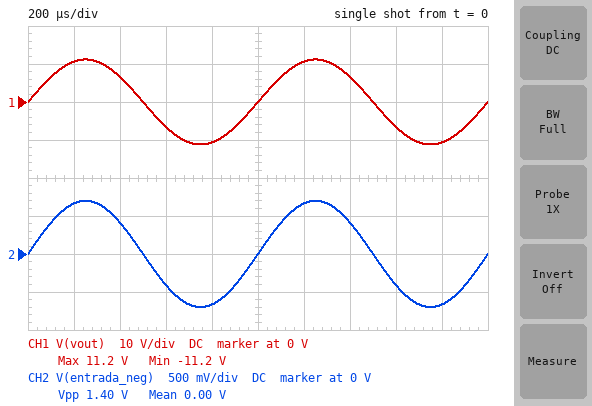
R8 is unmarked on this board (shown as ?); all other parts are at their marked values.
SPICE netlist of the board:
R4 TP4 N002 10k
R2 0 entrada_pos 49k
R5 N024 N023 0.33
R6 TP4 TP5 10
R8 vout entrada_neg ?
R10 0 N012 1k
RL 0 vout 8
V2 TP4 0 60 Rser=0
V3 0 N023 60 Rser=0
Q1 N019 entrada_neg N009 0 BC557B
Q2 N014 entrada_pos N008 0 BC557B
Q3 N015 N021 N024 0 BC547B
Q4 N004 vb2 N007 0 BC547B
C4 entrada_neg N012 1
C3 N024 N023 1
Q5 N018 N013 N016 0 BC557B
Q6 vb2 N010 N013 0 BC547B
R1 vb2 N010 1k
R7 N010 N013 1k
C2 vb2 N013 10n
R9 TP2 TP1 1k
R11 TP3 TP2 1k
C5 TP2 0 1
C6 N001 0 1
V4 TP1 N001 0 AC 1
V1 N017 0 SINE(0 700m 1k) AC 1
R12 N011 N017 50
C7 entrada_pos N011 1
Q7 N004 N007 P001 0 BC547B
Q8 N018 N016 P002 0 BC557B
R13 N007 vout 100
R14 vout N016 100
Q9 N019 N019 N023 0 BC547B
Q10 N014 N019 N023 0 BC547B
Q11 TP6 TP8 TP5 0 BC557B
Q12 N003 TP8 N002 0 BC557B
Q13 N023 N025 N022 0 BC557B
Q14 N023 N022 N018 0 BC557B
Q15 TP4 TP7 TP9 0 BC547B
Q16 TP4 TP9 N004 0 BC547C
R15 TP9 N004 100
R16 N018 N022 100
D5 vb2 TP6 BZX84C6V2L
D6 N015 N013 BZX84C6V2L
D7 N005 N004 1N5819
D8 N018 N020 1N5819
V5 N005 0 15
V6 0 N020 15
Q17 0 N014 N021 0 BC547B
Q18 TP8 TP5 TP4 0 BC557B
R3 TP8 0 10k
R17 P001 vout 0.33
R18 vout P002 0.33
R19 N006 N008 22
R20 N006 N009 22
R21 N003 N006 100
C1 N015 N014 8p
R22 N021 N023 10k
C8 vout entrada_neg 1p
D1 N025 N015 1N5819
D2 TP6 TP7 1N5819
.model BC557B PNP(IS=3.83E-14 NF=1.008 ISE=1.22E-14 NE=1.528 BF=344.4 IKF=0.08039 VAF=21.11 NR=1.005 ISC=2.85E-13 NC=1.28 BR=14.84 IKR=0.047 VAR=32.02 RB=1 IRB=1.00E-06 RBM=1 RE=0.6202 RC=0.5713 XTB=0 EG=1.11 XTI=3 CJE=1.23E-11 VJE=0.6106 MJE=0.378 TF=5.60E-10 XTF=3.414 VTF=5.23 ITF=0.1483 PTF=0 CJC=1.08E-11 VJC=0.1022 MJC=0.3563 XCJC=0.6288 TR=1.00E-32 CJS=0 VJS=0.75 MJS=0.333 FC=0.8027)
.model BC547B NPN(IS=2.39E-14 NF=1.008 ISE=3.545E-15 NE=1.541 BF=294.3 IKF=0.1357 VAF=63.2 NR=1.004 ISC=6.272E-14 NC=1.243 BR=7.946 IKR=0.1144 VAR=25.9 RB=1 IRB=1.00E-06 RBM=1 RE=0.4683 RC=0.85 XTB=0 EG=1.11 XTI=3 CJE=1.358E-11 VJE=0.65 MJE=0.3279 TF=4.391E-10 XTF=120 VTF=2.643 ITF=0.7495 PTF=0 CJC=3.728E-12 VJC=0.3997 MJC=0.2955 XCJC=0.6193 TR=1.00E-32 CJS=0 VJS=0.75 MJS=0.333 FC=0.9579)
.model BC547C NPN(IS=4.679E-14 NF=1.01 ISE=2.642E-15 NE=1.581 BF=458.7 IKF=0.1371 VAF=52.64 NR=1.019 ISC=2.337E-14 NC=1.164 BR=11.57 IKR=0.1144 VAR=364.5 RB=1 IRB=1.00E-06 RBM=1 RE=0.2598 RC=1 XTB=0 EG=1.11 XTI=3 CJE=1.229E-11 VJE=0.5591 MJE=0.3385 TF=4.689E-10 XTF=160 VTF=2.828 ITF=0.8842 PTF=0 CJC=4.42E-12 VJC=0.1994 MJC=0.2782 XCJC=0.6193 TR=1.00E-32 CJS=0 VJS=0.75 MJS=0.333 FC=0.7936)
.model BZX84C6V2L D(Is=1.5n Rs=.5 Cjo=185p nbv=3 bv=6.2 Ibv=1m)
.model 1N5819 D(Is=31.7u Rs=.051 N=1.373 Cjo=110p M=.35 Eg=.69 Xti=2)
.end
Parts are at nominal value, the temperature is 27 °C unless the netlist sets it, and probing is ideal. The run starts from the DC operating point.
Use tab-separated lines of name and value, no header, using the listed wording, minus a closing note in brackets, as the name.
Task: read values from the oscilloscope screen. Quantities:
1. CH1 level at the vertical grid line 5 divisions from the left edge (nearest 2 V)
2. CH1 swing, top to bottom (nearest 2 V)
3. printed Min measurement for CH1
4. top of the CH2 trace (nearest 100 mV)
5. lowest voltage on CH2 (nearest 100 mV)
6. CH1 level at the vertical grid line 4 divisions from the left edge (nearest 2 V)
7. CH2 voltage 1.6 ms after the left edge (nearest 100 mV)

CH1 level at the vertical grid line 5 divisions from the left edge	0 V
CH1 swing, top to bottom	22 V
printed Min measurement for CH1	-11.2 V
top of the CH2 trace	700 mV
lowest voltage on CH2	-700 mV
CH1 level at the vertical grid line 4 divisions from the left edge	-10 V
CH2 voltage 1.6 ms after the left edge	-400 mV
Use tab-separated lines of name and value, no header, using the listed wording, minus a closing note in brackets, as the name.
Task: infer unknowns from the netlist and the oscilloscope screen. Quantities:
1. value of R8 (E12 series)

value of R8	15 kΩ
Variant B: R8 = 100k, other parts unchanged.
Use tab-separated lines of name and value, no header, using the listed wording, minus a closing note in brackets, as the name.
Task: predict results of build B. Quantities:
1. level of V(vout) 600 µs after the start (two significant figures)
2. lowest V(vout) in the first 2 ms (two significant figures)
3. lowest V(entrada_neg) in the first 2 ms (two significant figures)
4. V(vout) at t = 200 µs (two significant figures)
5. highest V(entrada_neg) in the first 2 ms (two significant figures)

level of V(vout) 600 µs after the start	-41 V
lowest V(vout) in the first 2 ms	-45 V
lowest V(entrada_neg) in the first 2 ms	-440 mV
V(vout) at t = 200 µs	45 V
highest V(entrada_neg) in the first 2 ms	450 mV
